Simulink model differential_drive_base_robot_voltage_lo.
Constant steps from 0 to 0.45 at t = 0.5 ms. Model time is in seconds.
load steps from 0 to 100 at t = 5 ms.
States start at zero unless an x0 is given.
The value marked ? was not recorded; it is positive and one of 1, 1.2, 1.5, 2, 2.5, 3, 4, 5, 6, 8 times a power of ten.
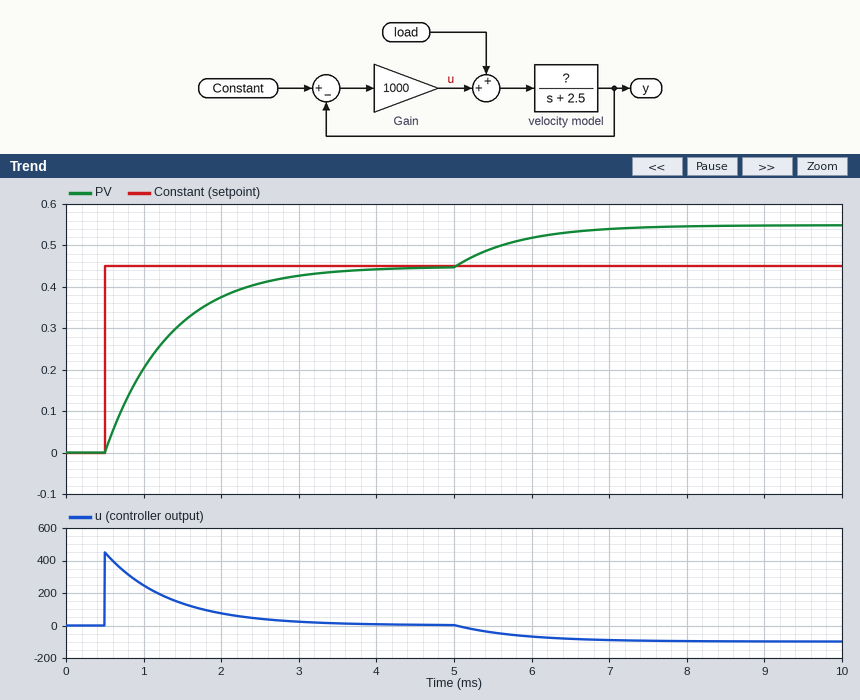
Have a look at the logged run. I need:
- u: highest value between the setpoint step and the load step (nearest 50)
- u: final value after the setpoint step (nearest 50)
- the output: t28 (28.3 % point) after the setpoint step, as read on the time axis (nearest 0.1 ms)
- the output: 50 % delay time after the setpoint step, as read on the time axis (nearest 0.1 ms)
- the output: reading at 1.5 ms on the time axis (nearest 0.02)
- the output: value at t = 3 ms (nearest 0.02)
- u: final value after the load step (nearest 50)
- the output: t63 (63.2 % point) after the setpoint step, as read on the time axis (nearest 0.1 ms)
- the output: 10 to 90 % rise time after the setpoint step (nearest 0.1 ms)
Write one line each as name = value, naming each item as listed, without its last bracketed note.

u: highest value between the setpoint step and the load step = 450
u: final value after the setpoint step = 0
the output: t28 (28.3 % point) after the setpoint step, as read on the time axis = 0.8 ms
the output: 50 % delay time after the setpoint step, as read on the time axis = 1.1 ms
the output: reading at 1.5 ms on the time axis = 0.32
the output: value at t = 3 ms = 0.42
u: final value after the load step = -100
the output: t63 (63.2 % point) after the setpoint step, as read on the time axis = 1.3 ms
the output: 10 to 90 % rise time after the setpoint step = 1.8 ms
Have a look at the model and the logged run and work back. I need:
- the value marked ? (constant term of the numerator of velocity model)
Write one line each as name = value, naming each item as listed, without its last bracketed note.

the value marked ? = 1.2
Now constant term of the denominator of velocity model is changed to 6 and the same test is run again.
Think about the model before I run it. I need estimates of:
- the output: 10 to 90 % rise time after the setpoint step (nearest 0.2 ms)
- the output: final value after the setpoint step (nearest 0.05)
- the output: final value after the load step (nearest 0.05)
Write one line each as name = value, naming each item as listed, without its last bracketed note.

the output: 10 to 90 % rise time after the setpoint step = 1.8 ms
the output: final value after the setpoint step = 0.45
the output: final value after the load step = 0.55
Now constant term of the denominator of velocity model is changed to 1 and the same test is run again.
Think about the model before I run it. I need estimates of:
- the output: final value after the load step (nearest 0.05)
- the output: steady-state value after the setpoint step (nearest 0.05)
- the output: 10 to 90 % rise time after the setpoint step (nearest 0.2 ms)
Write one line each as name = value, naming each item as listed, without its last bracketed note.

the output: final value after the load step = 0.55
the output: steady-state value after the setpoint step = 0.45
the output: 10 to 90 % rise time after the setpoint step = 1.8 ms
